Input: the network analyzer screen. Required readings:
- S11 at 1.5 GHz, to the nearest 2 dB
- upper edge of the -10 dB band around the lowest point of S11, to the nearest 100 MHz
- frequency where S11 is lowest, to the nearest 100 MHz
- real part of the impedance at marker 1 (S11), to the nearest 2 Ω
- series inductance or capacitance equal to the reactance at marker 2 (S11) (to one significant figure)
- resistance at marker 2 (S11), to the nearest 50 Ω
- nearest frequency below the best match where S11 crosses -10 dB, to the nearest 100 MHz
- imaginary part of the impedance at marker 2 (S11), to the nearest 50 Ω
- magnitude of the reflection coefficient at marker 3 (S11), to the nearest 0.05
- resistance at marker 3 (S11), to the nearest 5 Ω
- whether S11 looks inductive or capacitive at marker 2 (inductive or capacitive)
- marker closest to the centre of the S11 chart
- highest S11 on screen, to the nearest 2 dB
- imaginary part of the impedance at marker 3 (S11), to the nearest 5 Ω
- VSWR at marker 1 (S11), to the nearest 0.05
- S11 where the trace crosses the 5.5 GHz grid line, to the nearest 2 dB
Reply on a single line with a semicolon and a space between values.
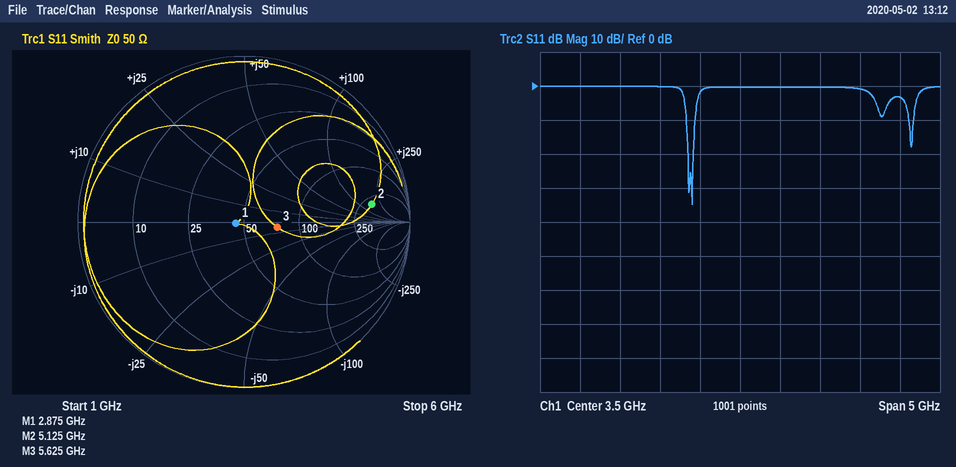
0 dB; 2.9 GHz; 2.9 GHz; 46 Ω; 5 nH; 300 Ω; 2.8 GHz; +150 Ω; 0.20; 75 Ω; inductive; marker 1; 0 dB; -5 Ω; 1.10; -4 dB
